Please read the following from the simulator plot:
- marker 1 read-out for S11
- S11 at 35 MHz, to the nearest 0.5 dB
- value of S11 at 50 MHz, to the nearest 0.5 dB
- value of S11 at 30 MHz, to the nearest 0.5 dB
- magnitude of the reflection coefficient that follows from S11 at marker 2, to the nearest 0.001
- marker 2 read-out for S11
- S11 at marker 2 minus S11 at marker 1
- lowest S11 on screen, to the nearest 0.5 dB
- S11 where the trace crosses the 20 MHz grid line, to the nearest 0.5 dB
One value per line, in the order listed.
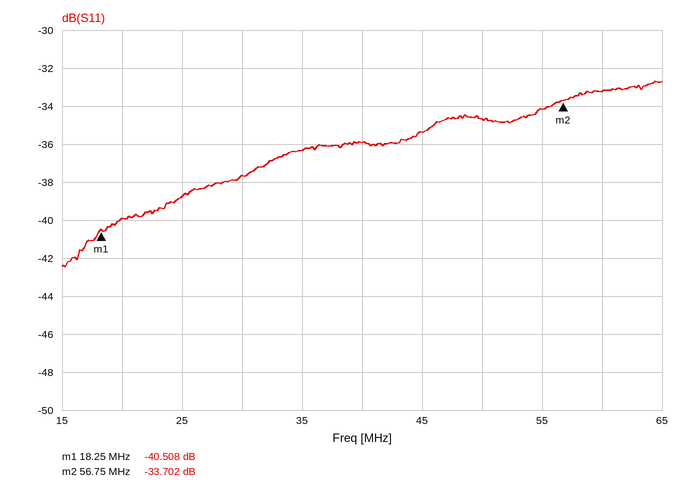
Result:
-40.508 dB
-36.5 dB
-34.5 dB
-37.5 dB
0.021
-33.702 dB
6.806 dB
-42.5 dB
-40.0 dB
